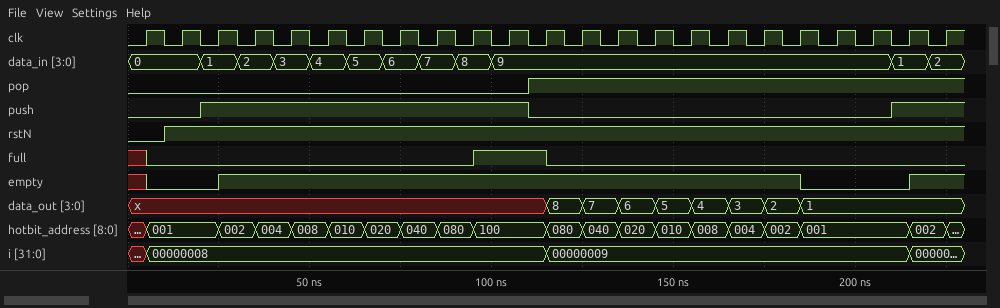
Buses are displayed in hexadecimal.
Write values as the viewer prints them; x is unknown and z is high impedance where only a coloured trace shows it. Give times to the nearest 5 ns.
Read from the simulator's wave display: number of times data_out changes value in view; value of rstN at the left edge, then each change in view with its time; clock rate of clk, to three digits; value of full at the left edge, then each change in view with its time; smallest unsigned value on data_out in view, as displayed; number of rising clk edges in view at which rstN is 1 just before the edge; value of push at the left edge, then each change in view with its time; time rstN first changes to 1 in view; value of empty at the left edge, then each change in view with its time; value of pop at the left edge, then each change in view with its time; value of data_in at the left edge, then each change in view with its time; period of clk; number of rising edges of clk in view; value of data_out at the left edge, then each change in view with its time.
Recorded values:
8
0, 1 at 10 ns
100 MHz
x, 0 at 5 ns, 1 at 95 ns, 0 at 115 ns
1
22
0, 1 at 20 ns, 0 at 110 ns, 1 at 210 ns
10 ns
x, 0 at 5 ns, 1 at 25 ns, 0 at 185 ns, 1 at 215 ns
0, 1 at 110 ns
0, 1 at 20 ns, 2 at 30 ns, 3 at 40 ns, 4 at 50 ns, 5 at 60 ns, 6 at 70 ns, 7 at 80 ns, 8 at 90 ns, 9 at 100 ns, 1 at 210 ns, 2 at 220 ns
10 ns
23
x, 8 at 115 ns, 7 at 125 ns, 6 at 135 ns, 5 at 145 ns, 4 at 155 ns, 3 at 165 ns, 2 at 175 ns, 1 at 185 ns
